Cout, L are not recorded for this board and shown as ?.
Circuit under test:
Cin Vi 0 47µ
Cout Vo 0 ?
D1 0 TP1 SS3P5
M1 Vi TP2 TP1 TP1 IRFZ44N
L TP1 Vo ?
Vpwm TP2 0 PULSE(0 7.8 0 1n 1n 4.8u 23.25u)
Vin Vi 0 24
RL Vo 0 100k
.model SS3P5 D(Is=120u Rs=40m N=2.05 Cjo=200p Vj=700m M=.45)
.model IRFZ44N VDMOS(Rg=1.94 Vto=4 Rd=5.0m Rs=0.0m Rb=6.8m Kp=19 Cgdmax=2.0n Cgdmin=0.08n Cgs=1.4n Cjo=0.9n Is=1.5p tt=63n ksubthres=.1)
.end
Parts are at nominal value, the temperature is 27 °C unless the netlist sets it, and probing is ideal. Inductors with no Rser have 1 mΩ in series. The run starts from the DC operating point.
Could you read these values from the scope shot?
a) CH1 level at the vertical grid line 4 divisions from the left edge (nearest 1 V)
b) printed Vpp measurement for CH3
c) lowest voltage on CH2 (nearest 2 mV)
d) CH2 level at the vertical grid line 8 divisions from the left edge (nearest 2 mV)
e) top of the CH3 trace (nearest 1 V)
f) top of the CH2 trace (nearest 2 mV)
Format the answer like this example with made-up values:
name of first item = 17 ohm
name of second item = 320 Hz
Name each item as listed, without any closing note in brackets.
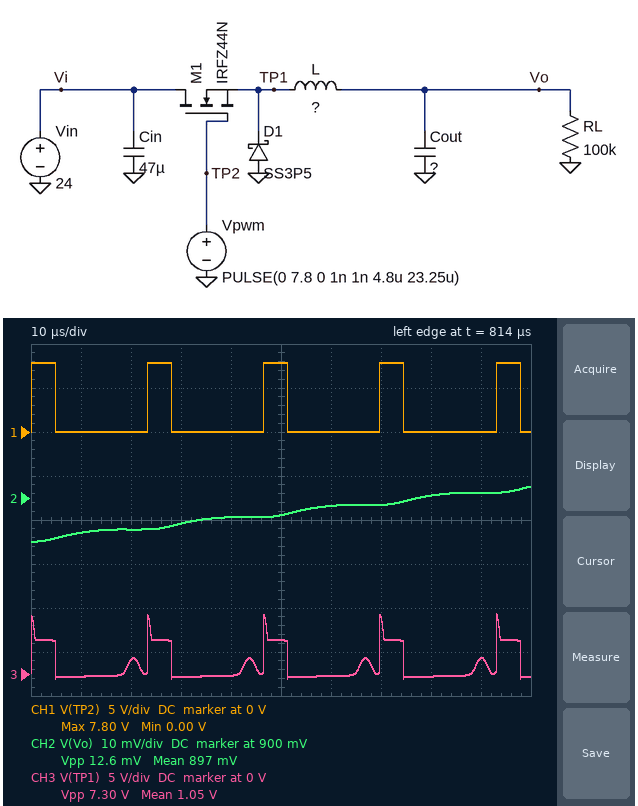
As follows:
CH1 level at the vertical grid line 4 divisions from the left edge = 0 V
printed Vpp measurement for CH3 = 7.30 V
lowest voltage on CH2 = 890 mV
CH2 level at the vertical grid line 8 divisions from the left edge = 900 mV
top of the CH3 trace = 7 V
top of the CH2 trace = 902 mV
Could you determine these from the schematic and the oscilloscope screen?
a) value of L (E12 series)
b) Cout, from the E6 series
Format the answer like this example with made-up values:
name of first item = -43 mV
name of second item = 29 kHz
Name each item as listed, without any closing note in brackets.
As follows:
value of L = 330 µH
Cout, from the E6 series = 150 µF
